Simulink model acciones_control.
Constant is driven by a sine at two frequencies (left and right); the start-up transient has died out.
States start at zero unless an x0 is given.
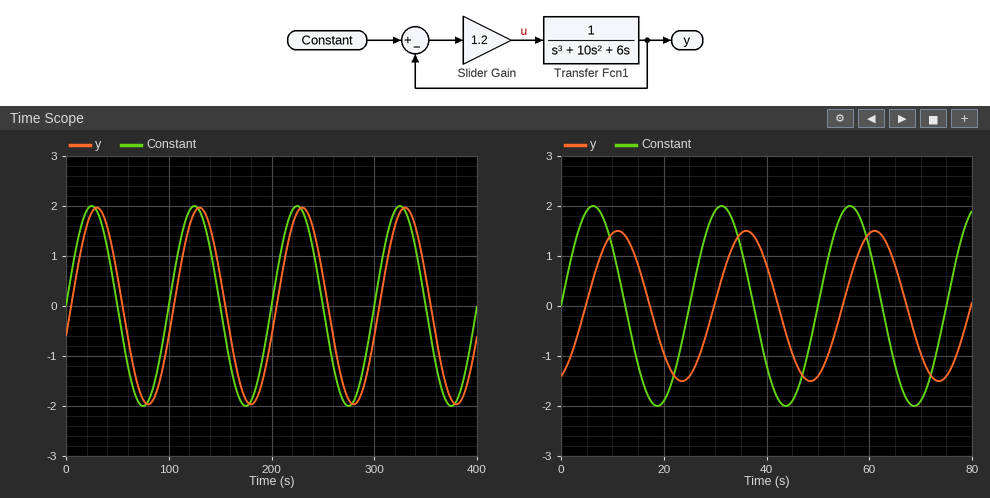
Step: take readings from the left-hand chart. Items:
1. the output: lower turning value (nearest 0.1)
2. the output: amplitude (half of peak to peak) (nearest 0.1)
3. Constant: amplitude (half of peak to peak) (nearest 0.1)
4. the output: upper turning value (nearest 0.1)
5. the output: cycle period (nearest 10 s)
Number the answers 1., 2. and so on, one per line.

1. -2.0
2. 2.0
3. 2.0
4. 2.0
5. 100 s
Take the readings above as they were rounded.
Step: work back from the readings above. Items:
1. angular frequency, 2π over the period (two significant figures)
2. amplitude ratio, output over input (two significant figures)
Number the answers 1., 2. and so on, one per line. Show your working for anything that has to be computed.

1. 2π / 100 = 0.063 rad/s
2. 2 / 2 = 1.0
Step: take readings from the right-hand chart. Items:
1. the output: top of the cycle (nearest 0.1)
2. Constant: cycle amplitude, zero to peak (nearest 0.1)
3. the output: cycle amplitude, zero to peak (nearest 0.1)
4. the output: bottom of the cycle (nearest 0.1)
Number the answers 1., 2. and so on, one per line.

1. 1.5
2. 2.0
3. 1.5
4. -1.5
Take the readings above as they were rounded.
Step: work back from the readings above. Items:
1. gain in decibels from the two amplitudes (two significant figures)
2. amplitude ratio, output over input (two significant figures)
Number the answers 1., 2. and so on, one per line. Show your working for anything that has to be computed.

1. 20 log10(1.5 / 2) = -2.5 dB
2. 1.5 / 2 = 0.75
